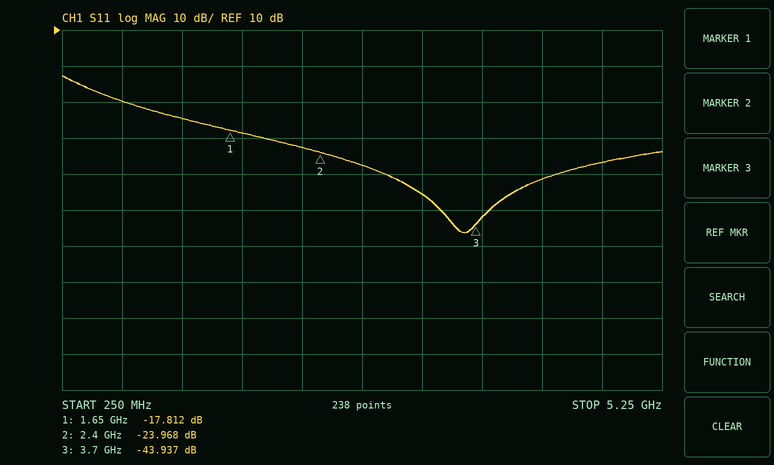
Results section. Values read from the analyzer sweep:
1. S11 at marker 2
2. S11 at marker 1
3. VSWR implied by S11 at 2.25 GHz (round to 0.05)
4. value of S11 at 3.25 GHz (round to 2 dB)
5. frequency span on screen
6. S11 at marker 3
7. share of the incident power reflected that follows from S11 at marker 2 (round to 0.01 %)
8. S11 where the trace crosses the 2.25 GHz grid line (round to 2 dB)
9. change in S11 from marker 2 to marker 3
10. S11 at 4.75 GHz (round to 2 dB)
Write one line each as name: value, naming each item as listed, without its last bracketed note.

S11 at marker 2: -23.968 dB
S11 at marker 1: -17.812 dB
VSWR implied by S11 at 2.25 GHz: 1.15
value of S11 at 3.25 GHz: -36 dB
frequency span on screen: 5 GHz
S11 at marker 3: -43.937 dB
share of the incident power reflected that follows from S11 at marker 2: 0.40 %
S11 where the trace crosses the 2.25 GHz grid line: -22 dB
change in S11 from marker 2 to marker 3: -19.969 dB
S11 at 4.75 GHz: -26 dB
